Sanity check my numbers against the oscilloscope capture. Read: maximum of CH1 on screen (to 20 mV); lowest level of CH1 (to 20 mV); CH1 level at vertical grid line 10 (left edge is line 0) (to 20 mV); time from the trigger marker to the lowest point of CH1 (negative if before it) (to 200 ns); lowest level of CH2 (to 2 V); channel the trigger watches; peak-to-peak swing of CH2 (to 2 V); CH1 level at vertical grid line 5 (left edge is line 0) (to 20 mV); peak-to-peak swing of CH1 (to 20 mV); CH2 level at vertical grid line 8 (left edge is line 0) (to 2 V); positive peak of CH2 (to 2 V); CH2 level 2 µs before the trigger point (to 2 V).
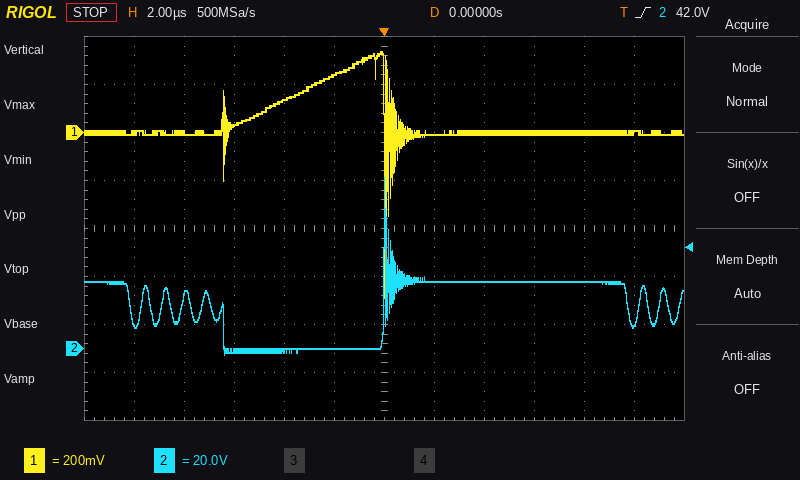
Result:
340 mV
-680 mV
0 mV
0.0 µs
-2 V
CH2
74 V
240 mV
1.02 V
28 V
72 V
0 V
